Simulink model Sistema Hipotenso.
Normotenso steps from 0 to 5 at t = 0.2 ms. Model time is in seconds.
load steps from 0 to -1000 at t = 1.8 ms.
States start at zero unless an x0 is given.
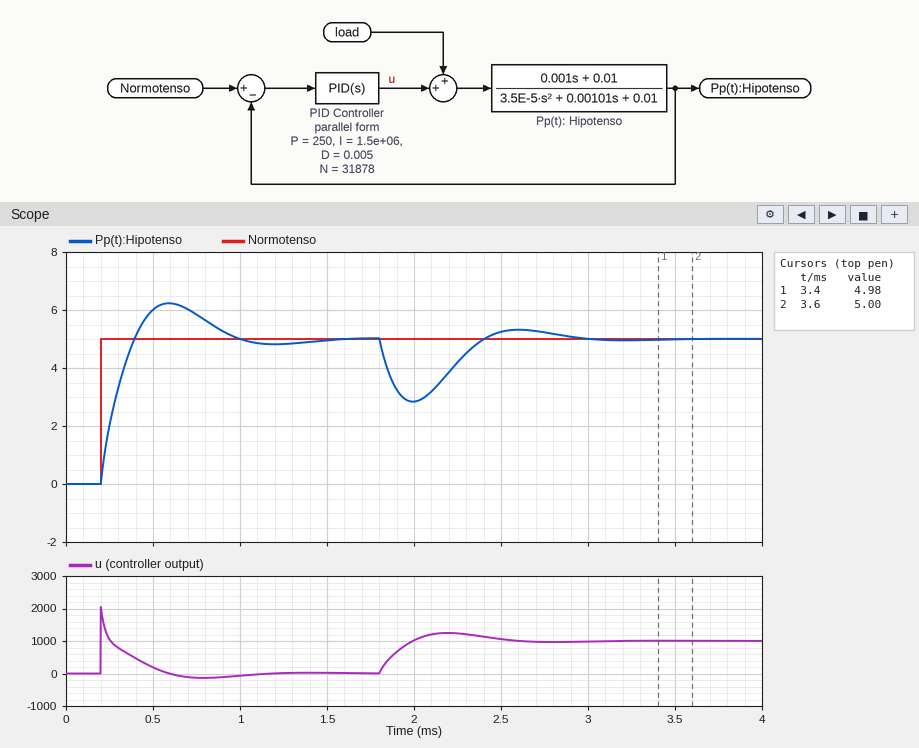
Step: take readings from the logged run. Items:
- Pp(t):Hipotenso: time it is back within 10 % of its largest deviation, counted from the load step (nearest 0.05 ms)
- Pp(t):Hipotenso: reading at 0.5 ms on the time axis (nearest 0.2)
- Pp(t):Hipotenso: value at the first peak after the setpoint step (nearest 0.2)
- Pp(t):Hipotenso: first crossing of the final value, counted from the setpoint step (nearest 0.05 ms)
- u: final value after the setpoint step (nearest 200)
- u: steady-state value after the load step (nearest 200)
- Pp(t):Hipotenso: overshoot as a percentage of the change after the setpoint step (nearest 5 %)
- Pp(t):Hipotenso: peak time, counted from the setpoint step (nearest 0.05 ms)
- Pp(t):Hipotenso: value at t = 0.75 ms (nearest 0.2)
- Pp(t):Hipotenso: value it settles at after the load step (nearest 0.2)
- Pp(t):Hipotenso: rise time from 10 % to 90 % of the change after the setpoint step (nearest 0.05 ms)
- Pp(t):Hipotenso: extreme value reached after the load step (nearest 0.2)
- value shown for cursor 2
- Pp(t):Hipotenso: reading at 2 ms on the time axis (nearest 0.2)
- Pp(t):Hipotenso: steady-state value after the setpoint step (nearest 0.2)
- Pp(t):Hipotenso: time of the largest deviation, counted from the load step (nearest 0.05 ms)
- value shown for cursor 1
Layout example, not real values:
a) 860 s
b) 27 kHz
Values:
a) 0.95 ms
b) 6.0
c) 6.2
d) 0.20 ms
e) 0
f) 1000
g) 25 %
h) 0.40 ms
i) 5.8
j) 5.0
k) 0.15 ms
l) 2.8
m) 5.00
n) 2.8
o) 5.0
p) 0.20 ms
q) 4.98
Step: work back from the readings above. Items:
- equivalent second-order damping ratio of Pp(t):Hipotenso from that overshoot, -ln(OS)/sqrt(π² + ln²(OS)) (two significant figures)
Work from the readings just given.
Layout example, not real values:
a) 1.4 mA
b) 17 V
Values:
a) 0.40
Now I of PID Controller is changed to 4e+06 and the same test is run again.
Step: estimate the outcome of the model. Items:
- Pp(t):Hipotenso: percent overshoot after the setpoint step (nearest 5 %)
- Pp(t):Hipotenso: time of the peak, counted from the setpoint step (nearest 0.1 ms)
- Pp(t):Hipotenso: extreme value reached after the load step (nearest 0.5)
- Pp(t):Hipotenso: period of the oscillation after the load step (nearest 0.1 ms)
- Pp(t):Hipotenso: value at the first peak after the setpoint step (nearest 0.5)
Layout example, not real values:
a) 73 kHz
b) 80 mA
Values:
a) 35 %
b) 0.3 ms
c) 3.5
d) 0.7 ms
e) 7.0
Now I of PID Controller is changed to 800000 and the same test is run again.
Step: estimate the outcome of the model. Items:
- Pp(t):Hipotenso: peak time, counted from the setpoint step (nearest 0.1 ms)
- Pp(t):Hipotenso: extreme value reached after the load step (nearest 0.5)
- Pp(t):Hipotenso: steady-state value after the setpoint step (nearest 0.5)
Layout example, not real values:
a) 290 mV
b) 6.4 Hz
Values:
a) 0.5 ms
b) 2.5
c) 5.0
